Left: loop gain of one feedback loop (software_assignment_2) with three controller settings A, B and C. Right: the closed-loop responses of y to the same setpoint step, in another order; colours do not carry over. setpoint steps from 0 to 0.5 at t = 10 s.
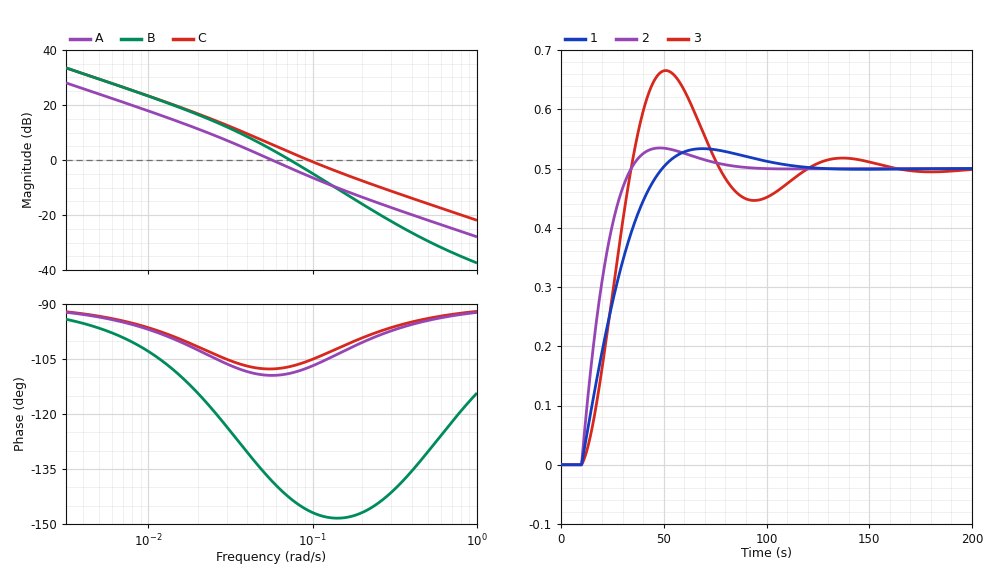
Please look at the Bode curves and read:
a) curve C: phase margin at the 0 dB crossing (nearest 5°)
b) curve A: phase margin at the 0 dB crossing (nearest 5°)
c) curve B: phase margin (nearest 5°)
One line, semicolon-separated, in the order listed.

75°; 70°; 35°
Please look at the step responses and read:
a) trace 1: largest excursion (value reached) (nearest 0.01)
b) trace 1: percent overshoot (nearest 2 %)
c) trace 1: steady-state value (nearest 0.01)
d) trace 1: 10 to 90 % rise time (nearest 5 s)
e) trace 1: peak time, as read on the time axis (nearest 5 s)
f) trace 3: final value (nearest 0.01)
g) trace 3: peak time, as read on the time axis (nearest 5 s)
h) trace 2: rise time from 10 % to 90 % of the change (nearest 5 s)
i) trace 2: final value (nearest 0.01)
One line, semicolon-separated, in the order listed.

0.53; 6 %; 0.50; 30 s; 70 s; 0.50; 50 s; 15 s; 0.50
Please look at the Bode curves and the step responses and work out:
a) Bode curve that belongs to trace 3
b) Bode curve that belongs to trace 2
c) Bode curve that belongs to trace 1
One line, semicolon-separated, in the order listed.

B; C; A
